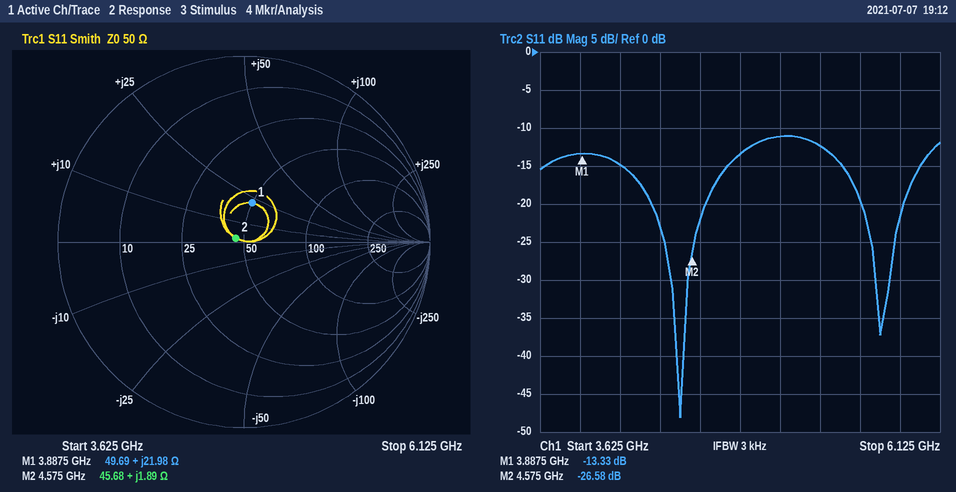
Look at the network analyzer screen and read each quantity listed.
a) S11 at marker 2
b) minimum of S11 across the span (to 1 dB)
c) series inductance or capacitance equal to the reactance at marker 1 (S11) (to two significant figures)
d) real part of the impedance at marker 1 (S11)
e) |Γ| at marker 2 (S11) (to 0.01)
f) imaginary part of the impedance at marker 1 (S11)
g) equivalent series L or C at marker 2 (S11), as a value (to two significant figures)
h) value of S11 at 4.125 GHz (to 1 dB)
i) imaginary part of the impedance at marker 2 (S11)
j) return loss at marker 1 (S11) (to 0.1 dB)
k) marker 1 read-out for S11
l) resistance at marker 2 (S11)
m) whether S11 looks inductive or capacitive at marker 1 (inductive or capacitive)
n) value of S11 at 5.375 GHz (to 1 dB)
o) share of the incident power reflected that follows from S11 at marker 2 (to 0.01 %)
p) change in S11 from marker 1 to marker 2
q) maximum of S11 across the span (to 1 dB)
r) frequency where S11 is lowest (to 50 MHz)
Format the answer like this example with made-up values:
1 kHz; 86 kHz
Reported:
-26.58 dB; -48 dB; 900 pH; 49.69 Ω; 0.05; +21.98 Ω; 66 pH; -15 dB; +1.89 Ω; 13.3 dB; -13.33 dB; 45.68 Ω; inductive; -12 dB; 0.22 %; -13.25 dB; -11 dB; 4.50 GHz
